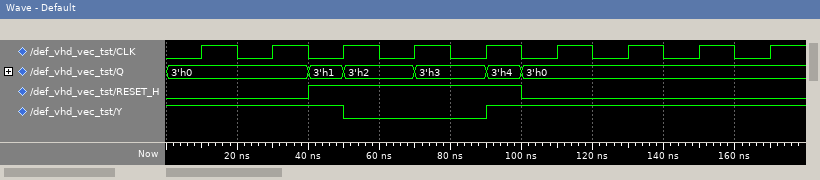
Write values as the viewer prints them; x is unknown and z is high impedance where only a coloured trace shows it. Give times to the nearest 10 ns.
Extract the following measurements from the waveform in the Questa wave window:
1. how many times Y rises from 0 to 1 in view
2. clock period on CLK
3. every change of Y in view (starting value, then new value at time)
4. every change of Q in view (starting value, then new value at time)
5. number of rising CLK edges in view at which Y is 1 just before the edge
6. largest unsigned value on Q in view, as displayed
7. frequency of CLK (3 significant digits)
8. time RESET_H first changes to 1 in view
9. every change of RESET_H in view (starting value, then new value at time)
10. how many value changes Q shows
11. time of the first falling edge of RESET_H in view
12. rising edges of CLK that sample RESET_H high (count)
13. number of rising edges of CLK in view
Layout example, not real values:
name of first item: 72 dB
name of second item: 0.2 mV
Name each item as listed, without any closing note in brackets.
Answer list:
how many times Y rises from 0 to 1 in view: 1
clock period on CLK: 20 ns
every change of Y in view: 1, 0 at 50 ns, 1 at 90 ns
every change of Q in view: 3'h0, 3'h1 at 40 ns, 3'h2 at 50 ns, 3'h3 at 70 ns, 3'h4 at 90 ns, 3'h0 at 100 ns
number of rising CLK edges in view at which Y is 1 just before the edge: 7
largest unsigned value on Q in view, as displayed: 3'h4
frequency of CLK: 50.0 MHz
time RESET_H first changes to 1 in view: 40 ns
every change of RESET_H in view: 0, 1 at 40 ns, 0 at 100 ns
how many value changes Q shows: 5
time of the first falling edge of RESET_H in view: 100 ns
rising edges of CLK that sample RESET_H high: 3
number of rising edges of CLK in view: 9
